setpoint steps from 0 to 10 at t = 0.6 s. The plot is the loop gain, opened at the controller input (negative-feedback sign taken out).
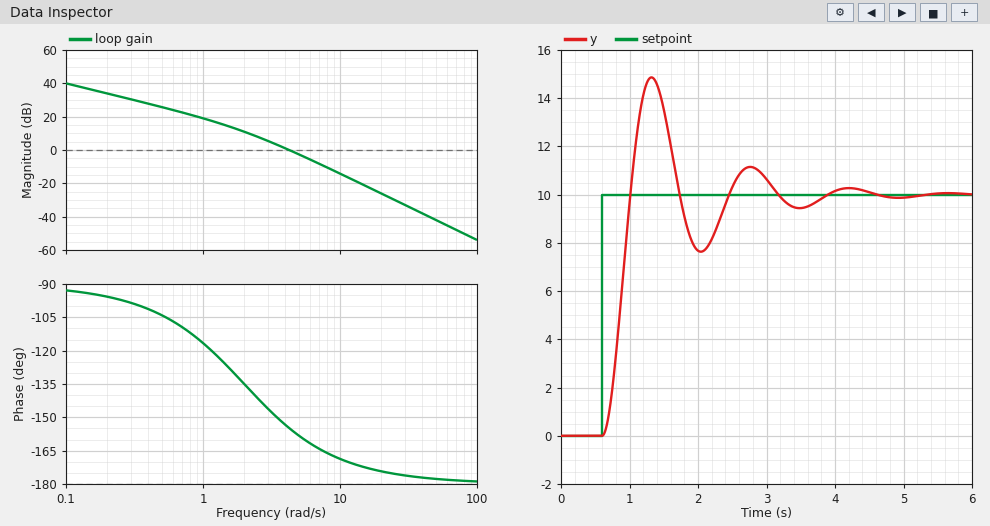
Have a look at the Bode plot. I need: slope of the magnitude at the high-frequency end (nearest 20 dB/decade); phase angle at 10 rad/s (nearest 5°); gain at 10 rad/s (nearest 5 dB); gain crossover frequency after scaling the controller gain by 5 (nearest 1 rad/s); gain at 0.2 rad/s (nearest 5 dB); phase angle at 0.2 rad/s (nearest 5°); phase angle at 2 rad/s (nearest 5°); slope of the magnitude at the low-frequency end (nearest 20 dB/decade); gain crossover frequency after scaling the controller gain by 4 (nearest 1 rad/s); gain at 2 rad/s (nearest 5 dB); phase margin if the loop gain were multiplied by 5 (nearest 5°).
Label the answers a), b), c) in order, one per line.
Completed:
a) -40 dB/decade
b) -170°
c) -15 dB
d) 10 rad/s
e) 35 dB
f) -95°
g) -135°
h) -20 dB/decade
i) 9 rad/s
j) 10 dB
k) 10°
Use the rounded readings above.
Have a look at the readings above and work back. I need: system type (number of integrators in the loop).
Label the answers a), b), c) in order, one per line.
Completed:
a) 1
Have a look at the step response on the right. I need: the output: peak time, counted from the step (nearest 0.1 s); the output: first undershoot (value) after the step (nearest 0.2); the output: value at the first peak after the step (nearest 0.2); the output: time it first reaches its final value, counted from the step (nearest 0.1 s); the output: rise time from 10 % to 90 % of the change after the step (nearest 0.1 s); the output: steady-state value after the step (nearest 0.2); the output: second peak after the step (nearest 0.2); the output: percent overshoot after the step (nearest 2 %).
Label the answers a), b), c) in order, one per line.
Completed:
a) 0.7 s
b) 7.6
c) 14.8
d) 0.4 s
e) 0.3 s
f) 10.0
g) 11.2
h) 48 %
